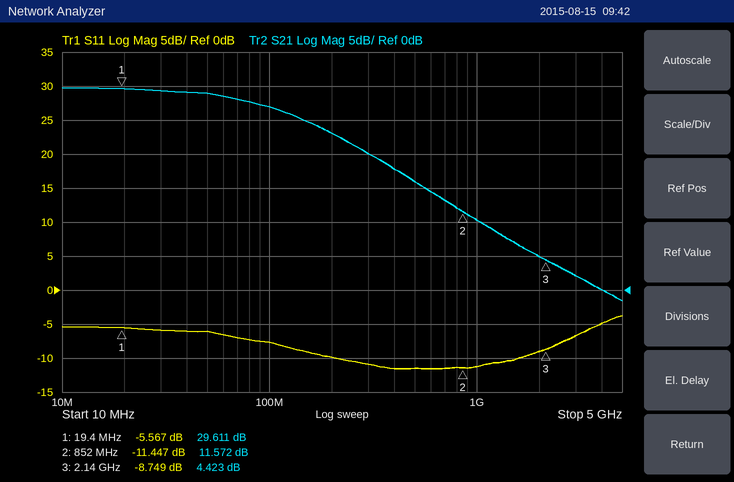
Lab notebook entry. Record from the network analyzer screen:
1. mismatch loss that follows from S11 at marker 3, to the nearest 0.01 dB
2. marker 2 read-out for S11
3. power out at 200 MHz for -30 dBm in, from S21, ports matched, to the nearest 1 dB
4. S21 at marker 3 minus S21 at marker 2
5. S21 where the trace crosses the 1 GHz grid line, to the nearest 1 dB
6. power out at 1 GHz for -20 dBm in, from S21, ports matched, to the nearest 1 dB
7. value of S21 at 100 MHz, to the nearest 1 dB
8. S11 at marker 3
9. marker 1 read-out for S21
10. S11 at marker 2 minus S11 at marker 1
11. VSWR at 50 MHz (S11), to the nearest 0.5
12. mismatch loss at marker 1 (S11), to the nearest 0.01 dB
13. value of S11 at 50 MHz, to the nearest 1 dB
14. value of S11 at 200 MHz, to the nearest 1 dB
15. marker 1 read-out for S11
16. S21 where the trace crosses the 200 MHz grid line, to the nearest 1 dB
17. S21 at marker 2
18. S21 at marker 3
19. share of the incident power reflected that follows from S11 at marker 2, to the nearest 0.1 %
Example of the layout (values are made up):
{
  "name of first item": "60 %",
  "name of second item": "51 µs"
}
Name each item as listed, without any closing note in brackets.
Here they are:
{
  "mismatch loss that follows from S11 at marker 3, to the nearest 0.01 dB": "0.62 dB",
  "marker 2 read-out for S11": "-11.447 dB",
  "power out at 200 MHz for -30 dBm in, from S21, ports matched, to the nearest 1 dB": "-7 dBm",
  "S21 at marker 3 minus S21 at marker 2": "-7.149 dB",
  "S21 where the trace crosses the 1 GHz grid line, to the nearest 1 dB": "10 dB",
  "power out at 1 GHz for -20 dBm in, from S21, ports matched, to the nearest 1 dB": "-10 dBm",
  "value of S21 at 100 MHz, to the nearest 1 dB": "27 dB",
  "S11 at marker 3": "-8.749 dB",
  "marker 1 read-out for S21": "29.611 dB",
  "S11 at marker 2 minus S11 at marker 1": "-5.880 dB",
  "VSWR at 50 MHz (S11), to the nearest 0.5": "3.0",
  "mismatch loss at marker 1 (S11), to the nearest 0.01 dB": "1.41 dB",
  "value of S11 at 50 MHz, to the nearest 1 dB": "-6 dB",
  "value of S11 at 200 MHz, to the nearest 1 dB": "-10 dB",
  "marker 1 read-out for S11": "-5.567 dB",
  "S21 where the trace crosses the 200 MHz grid line, to the nearest 1 dB": "23 dB",
  "S21 at marker 2": "11.572 dB",
  "S21 at marker 3": "4.423 dB",
  "share of the incident power reflected that follows from S11 at marker 2, to the nearest 0.1 %": "7.2 %"
}
